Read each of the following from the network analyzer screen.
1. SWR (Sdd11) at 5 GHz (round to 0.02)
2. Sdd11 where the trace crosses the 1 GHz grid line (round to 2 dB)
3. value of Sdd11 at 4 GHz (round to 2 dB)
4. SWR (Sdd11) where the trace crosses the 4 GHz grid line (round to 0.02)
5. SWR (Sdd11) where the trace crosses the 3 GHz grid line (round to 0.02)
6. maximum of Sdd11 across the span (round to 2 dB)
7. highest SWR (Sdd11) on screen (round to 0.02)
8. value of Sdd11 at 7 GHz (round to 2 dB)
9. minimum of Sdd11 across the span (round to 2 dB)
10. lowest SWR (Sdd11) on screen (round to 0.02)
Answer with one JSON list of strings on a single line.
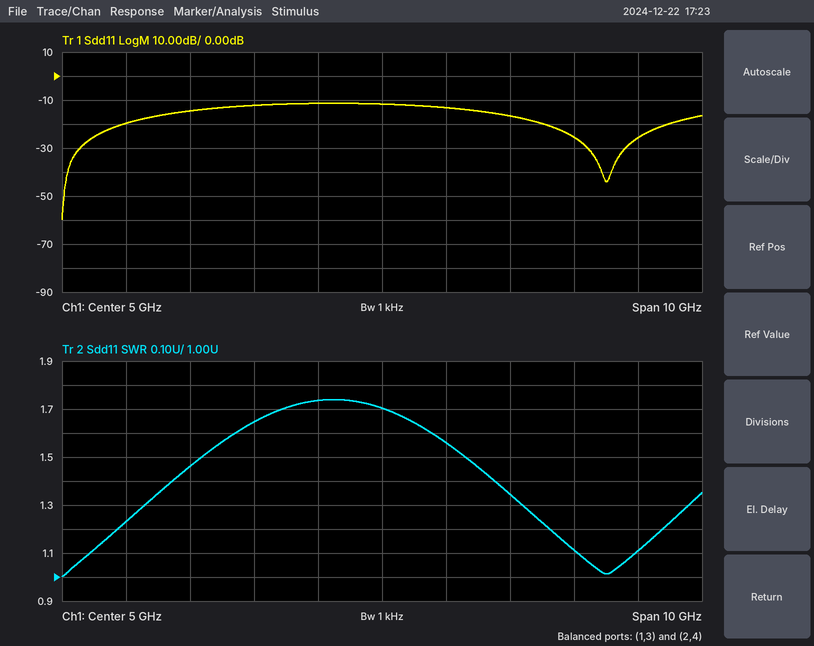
["1.70", "-20 dB", "-12 dB", "1.74", "1.64", "-12 dB", "1.74", "-16 dB", "-60 dB", "1.00"]
